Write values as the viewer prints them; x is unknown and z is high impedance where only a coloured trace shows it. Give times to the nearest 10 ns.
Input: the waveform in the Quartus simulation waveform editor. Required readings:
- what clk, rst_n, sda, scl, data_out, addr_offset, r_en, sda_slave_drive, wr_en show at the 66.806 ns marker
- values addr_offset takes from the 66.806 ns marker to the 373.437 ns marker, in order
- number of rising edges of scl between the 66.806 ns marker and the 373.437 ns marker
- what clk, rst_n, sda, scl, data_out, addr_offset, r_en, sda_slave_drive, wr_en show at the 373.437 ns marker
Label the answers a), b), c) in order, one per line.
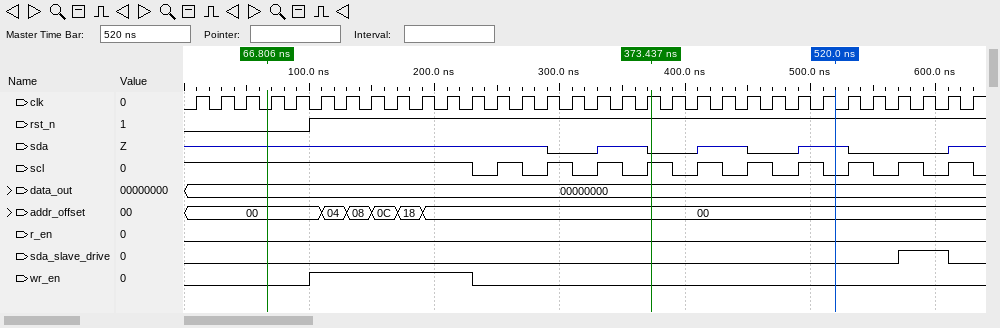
a) clk=0, rst_n=0, sda=z, scl=1, data_out=00000000, addr_offset=00, r_en=0, sda_slave_drive=0, wr_en=0
b) 00, 04, 08, 0C, 18, 00
c) 4
d) clk=1, rst_n=1, sda=0, scl=1, data_out=00000000, addr_offset=00, r_en=0, sda_slave_drive=0, wr_en=0
